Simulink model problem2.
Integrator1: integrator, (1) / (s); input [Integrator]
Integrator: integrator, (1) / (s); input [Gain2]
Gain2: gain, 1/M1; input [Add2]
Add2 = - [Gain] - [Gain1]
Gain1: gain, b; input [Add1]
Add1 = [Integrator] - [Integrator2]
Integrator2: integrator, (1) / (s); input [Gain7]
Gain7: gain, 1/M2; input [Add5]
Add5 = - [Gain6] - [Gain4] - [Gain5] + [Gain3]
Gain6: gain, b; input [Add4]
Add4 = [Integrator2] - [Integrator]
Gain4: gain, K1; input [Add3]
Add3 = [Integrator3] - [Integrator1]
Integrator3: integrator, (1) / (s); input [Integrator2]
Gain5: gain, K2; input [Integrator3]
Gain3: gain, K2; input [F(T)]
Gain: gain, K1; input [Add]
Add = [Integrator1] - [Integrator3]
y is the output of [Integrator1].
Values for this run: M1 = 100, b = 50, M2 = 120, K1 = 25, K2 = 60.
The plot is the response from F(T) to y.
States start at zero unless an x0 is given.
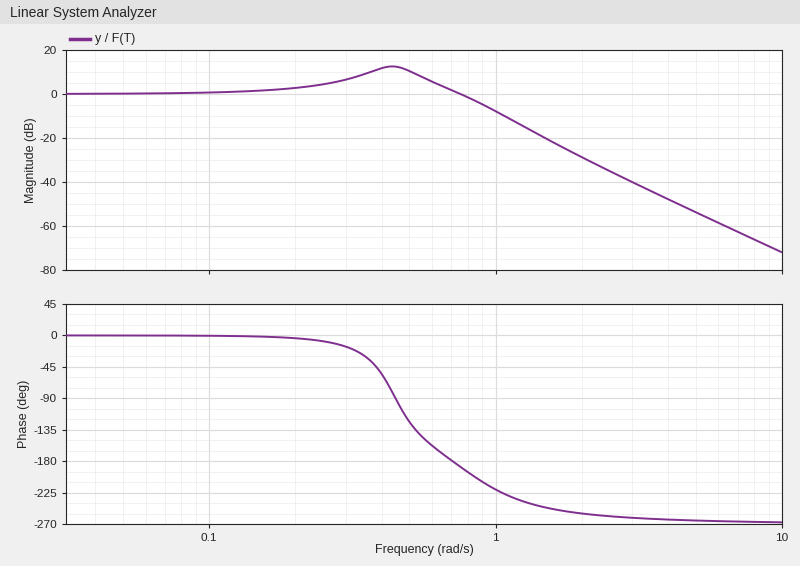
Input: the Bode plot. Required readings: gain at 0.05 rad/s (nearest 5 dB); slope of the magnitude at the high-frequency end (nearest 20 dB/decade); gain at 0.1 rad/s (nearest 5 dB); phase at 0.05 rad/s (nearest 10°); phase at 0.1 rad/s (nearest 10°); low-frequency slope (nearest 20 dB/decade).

0 dB
-60 dB/decade
0 dB
0°
0°
0 dB/decade
